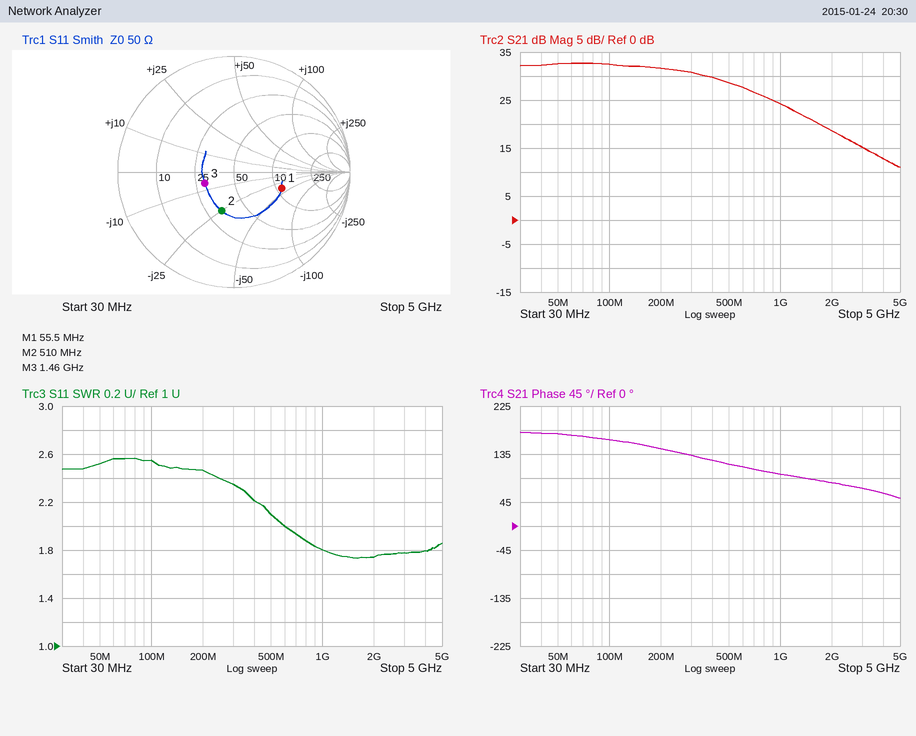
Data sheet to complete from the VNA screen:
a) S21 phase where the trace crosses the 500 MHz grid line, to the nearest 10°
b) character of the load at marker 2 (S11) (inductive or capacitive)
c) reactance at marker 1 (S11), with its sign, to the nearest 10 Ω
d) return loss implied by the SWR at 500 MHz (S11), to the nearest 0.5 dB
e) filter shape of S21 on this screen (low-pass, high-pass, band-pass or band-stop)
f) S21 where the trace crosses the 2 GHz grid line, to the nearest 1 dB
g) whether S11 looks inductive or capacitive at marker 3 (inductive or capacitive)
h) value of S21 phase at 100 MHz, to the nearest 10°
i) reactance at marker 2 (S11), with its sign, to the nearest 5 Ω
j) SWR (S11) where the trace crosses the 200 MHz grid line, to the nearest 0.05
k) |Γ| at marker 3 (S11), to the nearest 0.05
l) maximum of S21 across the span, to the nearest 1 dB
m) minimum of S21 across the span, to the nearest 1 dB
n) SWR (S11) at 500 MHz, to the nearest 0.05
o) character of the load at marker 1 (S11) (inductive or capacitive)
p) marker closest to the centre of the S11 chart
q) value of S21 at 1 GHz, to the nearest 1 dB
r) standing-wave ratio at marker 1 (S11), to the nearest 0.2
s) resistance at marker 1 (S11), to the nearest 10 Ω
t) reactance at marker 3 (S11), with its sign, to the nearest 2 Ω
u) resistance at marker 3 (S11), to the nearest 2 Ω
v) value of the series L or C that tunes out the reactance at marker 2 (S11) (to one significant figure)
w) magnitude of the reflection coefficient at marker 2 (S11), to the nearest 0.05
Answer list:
120°
capacitive
-40 Ω
9.0 dB
low-pass
19 dB
capacitive
160°
-25 Ω
2.45
0.25
33 dB
11 dB
2.10
capacitive
marker 3
24 dB
2.6
110 Ω
-6 Ω
30 Ω
8 nH
0.35
